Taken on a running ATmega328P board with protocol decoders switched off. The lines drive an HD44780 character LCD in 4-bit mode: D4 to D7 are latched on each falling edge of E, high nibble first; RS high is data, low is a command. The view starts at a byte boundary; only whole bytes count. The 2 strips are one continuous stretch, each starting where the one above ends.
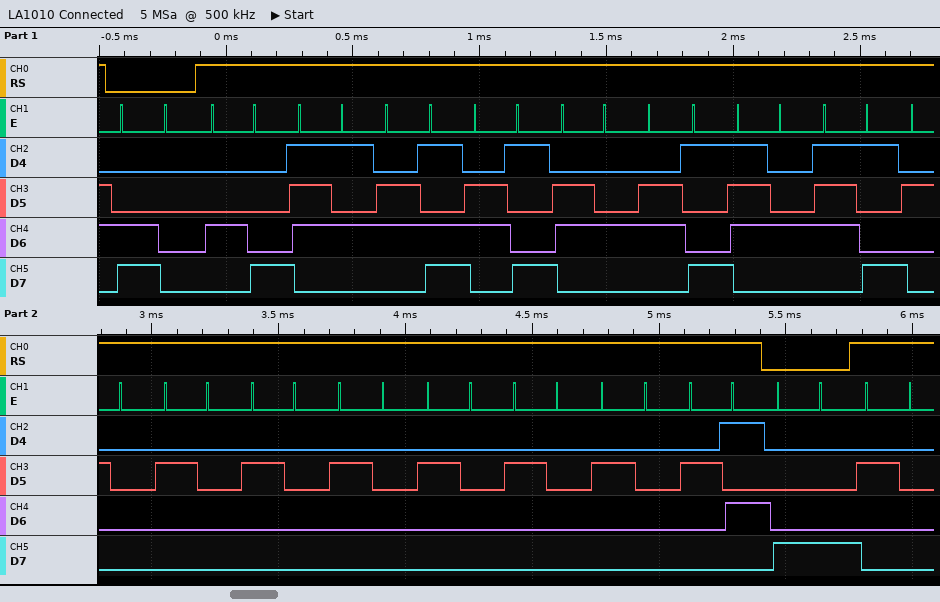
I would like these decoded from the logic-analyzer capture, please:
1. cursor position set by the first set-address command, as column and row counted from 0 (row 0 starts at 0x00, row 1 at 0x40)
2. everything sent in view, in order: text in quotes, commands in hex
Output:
column 0, row 1
0xC0 "Humidity       %" 0x88 " "
